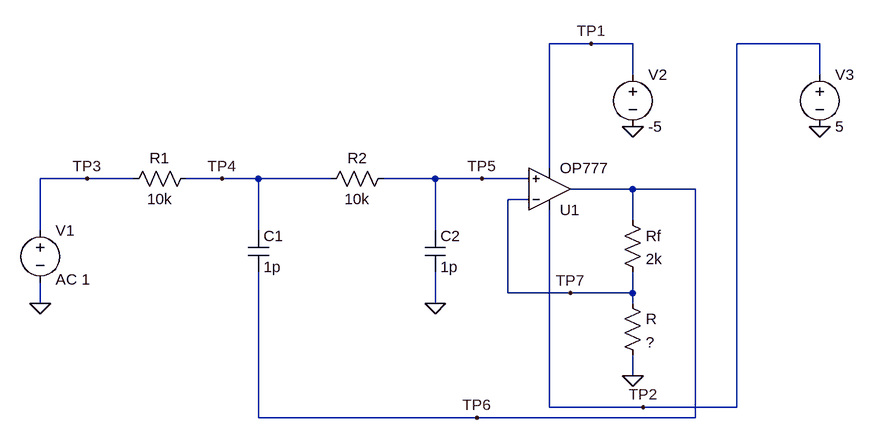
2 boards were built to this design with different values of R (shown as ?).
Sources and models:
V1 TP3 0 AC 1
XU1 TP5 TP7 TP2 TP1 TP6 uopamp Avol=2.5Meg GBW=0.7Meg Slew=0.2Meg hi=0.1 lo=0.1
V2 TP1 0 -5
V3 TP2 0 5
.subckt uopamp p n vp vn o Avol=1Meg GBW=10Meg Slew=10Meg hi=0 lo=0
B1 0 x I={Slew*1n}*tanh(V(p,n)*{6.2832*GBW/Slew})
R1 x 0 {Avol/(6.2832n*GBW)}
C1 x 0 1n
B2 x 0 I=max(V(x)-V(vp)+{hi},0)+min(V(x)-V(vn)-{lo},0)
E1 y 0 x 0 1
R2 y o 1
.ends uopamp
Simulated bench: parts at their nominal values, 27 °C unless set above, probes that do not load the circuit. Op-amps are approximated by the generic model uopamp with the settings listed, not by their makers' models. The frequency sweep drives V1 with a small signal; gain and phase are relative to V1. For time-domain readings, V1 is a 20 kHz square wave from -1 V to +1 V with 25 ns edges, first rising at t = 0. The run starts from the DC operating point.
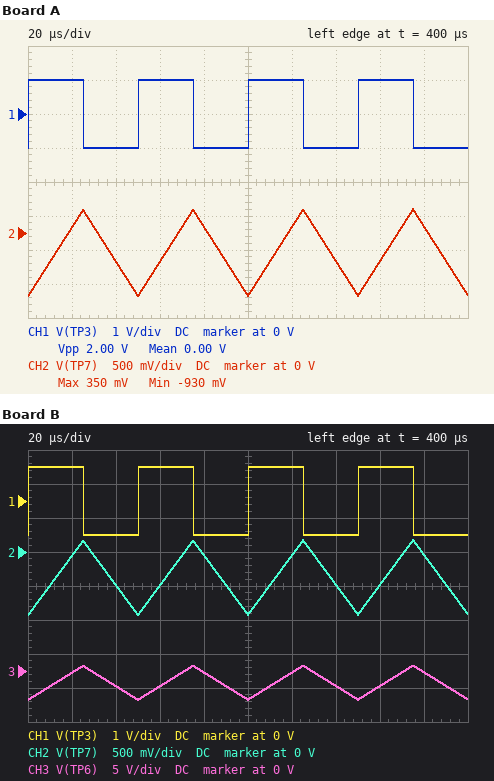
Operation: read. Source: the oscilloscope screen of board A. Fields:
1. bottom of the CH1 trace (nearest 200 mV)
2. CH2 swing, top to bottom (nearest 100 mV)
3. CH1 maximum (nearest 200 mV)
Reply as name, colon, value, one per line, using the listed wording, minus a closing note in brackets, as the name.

bottom of the CH1 trace: -1.0 V
CH2 swing, top to bottom: 1.3 V
CH1 maximum: 1.0 V
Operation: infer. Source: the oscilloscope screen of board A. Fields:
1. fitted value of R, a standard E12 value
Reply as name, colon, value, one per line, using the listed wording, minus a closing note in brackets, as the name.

fitted value of R, a standard E12 value: 680 Ω
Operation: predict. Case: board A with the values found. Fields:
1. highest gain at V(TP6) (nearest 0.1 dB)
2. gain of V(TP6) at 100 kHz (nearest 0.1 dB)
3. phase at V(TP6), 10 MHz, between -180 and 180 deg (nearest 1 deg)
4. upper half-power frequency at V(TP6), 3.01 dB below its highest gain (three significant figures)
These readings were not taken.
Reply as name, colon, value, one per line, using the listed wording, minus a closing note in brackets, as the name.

highest gain at V(TP6): 11.9 dB
gain of V(TP6) at 100 kHz: 10.8 dB
phase at V(TP6), 10 MHz, between -180 and 180 deg: -162 deg
upper half-power frequency at V(TP6), 3.01 dB below its highest gain: 186 kHz
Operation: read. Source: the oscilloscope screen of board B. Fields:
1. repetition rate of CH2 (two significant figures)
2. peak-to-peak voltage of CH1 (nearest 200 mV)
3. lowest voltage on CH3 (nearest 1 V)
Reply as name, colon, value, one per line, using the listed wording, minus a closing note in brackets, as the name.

repetition rate of CH2: 20 kHz
peak-to-peak voltage of CH1: 2.0 V
lowest voltage on CH3: -4 V
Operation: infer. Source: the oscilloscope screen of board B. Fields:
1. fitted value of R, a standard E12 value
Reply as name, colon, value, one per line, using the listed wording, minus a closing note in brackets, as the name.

fitted value of R, a standard E12 value: 560 Ω
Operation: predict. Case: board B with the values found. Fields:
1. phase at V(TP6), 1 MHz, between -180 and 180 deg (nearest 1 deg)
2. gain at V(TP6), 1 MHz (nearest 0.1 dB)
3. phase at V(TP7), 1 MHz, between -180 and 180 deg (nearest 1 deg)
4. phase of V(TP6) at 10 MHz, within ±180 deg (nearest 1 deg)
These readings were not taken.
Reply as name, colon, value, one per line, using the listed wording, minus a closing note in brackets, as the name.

phase at V(TP6), 1 MHz, between -180 and 180 deg: -92 deg
gain at V(TP6), 1 MHz: -2.9 dB
phase at V(TP7), 1 MHz, between -180 and 180 deg: -92 deg
phase of V(TP6) at 10 MHz, within ±180 deg: -163 deg
